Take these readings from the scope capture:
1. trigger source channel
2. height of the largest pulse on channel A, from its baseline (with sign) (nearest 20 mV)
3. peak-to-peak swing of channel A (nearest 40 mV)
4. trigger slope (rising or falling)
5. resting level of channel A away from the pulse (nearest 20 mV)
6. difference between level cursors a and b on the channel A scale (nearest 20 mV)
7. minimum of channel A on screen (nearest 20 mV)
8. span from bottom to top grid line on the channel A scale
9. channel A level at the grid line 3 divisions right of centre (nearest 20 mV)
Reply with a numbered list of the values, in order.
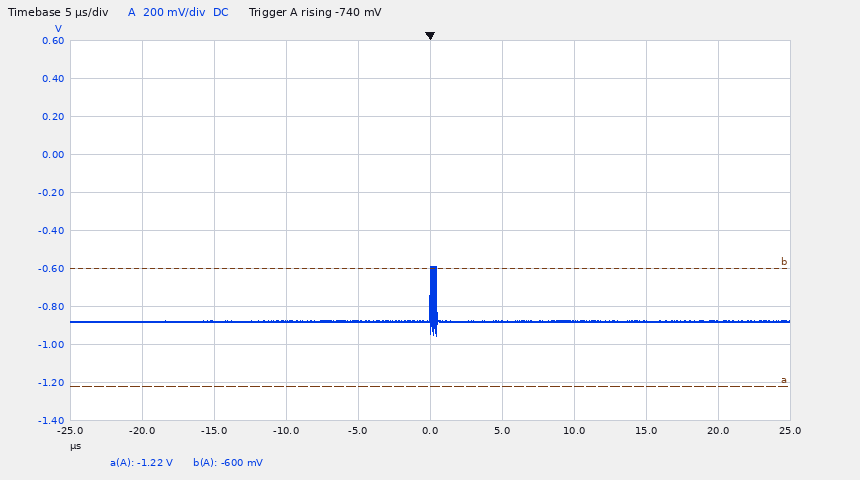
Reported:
1. channel A
2. +280 mV
3. 360 mV
4. rising
5. -880 mV
6. 620 mV
7. -960 mV
8. 2 V
9. -880 mV
